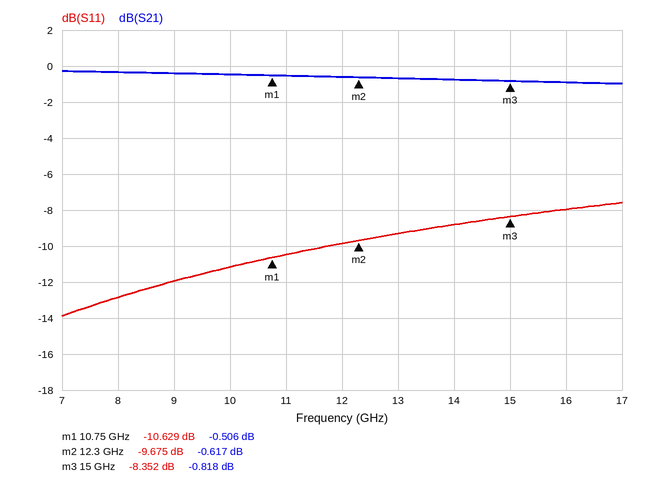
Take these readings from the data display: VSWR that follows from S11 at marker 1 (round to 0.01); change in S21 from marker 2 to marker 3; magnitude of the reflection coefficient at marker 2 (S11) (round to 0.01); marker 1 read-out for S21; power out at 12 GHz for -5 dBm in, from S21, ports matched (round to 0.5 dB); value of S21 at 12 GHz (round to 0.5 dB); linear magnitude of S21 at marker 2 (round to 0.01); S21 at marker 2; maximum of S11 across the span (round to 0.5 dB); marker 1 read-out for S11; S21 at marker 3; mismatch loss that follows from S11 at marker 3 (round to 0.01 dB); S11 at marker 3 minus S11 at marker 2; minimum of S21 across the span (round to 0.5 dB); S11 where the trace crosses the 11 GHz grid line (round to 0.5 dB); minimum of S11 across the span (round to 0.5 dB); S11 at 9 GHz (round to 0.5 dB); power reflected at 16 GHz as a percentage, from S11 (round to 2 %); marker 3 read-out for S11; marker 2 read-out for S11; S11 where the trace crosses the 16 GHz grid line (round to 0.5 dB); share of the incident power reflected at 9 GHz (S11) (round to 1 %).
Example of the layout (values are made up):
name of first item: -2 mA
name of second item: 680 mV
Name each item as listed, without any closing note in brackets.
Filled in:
VSWR that follows from S11 at marker 1: 1.83
change in S21 from marker 2 to marker 3: -0.201 dB
magnitude of the reflection coefficient at marker 2 (S11): 0.33
marker 1 read-out for S21: -0.506 dB
power out at 12 GHz for -5 dBm in, from S21, ports matched: -5.5 dBm
value of S21 at 12 GHz: -0.5 dB
linear magnitude of S21 at marker 2: 0.93
S21 at marker 2: -0.617 dB
maximum of S11 across the span: -7.5 dB
marker 1 read-out for S11: -10.629 dB
S21 at marker 3: -0.818 dB
mismatch loss that follows from S11 at marker 3: 0.69 dB
S11 at marker 3 minus S11 at marker 2: 1.323 dB
minimum of S21 across the span: -1.0 dB
S11 where the trace crosses the 11 GHz grid line: -10.5 dB
minimum of S11 across the span: -14.0 dB
S11 at 9 GHz: -12.0 dB
power reflected at 16 GHz as a percentage, from S11: 16 %
marker 3 read-out for S11: -8.352 dB
marker 2 read-out for S11: -9.675 dB
S11 where the trace crosses the 16 GHz grid line: -8.0 dB
share of the incident power reflected at 9 GHz (S11): 6 %
